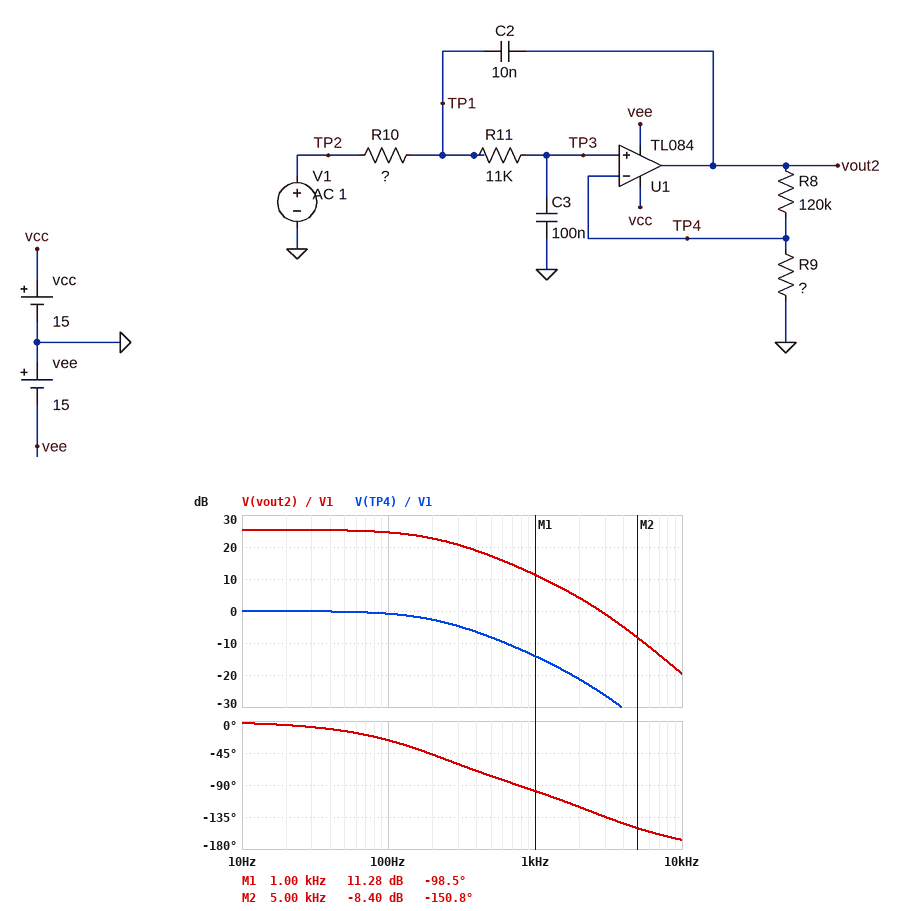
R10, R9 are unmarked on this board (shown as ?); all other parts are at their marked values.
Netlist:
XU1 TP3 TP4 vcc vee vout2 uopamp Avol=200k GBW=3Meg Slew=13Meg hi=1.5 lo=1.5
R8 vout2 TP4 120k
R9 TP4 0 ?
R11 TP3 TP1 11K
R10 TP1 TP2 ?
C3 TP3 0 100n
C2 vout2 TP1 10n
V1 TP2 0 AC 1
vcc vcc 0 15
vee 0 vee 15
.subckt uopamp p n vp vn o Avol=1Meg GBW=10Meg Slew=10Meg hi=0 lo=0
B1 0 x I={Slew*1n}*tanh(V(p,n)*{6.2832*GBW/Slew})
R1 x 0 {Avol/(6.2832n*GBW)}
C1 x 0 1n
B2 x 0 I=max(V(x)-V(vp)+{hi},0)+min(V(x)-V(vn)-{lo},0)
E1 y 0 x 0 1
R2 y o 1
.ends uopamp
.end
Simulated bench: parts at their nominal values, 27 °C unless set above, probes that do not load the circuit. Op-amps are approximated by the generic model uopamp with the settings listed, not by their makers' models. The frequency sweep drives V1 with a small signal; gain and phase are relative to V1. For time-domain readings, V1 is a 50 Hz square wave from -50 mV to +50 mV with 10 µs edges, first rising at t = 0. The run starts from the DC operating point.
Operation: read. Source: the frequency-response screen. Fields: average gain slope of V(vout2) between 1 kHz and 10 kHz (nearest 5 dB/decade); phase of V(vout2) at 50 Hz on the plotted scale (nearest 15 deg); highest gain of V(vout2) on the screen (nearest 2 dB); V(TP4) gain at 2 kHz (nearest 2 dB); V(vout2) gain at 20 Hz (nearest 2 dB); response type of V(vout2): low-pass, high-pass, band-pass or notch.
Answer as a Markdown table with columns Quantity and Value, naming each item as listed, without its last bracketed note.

| Quantity | Value |
|---|---|
| average gain slope of V(vout2) between 1 kHz and 10 kHz | -30 dB/decade |
| phase of V(vout2) at 50 Hz on the plotted scale | -15 deg |
| highest gain of V(vout2) on the screen | 26 dB |
| V(TP4) gain at 2 kHz | -22 dB |
| V(vout2) gain at 20 Hz | 26 dB |
| response type of V(vout2): low-pass, high-pass, band-pass or notch | low-pass |
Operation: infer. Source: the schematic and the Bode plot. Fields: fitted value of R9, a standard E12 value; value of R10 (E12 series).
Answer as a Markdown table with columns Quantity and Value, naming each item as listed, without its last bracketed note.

| Quantity | Value |
|---|---|
| fitted value of R9, a standard E12 value | 6.8 kΩ |
| value of R10 | 3.9 kΩ |
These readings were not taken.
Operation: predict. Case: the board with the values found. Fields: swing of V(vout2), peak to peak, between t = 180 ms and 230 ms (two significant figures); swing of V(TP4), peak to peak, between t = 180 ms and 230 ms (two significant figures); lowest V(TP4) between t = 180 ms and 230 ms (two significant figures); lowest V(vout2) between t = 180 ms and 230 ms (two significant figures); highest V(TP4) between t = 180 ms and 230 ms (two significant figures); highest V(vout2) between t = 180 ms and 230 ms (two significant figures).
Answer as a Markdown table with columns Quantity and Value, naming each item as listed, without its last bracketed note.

| Quantity | Value |
|---|---|
| swing of V(vout2), peak to peak, between t = 180 ms and 230 ms | 1.9 V |
| swing of V(TP4), peak to peak, between t = 180 ms and 230 ms | 100 mV |
| lowest V(TP4) between t = 180 ms and 230 ms | -50 mV |
| lowest V(vout2) between t = 180 ms and 230 ms | -930 mV |
| highest V(TP4) between t = 180 ms and 230 ms | 50 mV |
| highest V(vout2) between t = 180 ms and 230 ms | 930 mV |
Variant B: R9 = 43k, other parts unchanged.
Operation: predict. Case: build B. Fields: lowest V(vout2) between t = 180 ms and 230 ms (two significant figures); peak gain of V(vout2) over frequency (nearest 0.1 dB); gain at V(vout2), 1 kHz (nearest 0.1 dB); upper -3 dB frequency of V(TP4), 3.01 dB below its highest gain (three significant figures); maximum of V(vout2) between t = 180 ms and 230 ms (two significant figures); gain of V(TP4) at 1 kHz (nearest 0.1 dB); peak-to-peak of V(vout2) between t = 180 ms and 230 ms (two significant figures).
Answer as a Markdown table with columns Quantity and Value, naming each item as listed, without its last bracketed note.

| Quantity | Value |
|---|---|
| lowest V(vout2) between t = 180 ms and 230 ms | -190 mV |
| peak gain of V(vout2) over frequency | 11.6 dB |
| gain at V(vout2), 1 kHz | -7.2 dB |
| upper -3 dB frequency of V(TP4), 3.01 dB below its highest gain | 118 Hz |
| maximum of V(vout2) between t = 180 ms and 230 ms | 190 mV |
| gain of V(TP4) at 1 kHz | -18.8 dB |
| peak-to-peak of V(vout2) between t = 180 ms and 230 ms | 380 mV |
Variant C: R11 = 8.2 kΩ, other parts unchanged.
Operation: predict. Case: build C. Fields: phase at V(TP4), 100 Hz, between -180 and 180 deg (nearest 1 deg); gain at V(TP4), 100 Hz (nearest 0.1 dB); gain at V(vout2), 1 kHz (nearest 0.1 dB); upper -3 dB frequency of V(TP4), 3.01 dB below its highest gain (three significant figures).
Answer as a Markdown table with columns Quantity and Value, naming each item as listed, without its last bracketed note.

| Quantity | Value |
|---|---|
| phase at V(TP4), 100 Hz, between -180 and 180 deg | -18 deg |
| gain at V(TP4), 100 Hz | -0.3 dB |
| gain at V(vout2), 1 kHz | 15.1 dB |
| upper -3 dB frequency of V(TP4), 3.01 dB below its highest gain | 346 Hz |
